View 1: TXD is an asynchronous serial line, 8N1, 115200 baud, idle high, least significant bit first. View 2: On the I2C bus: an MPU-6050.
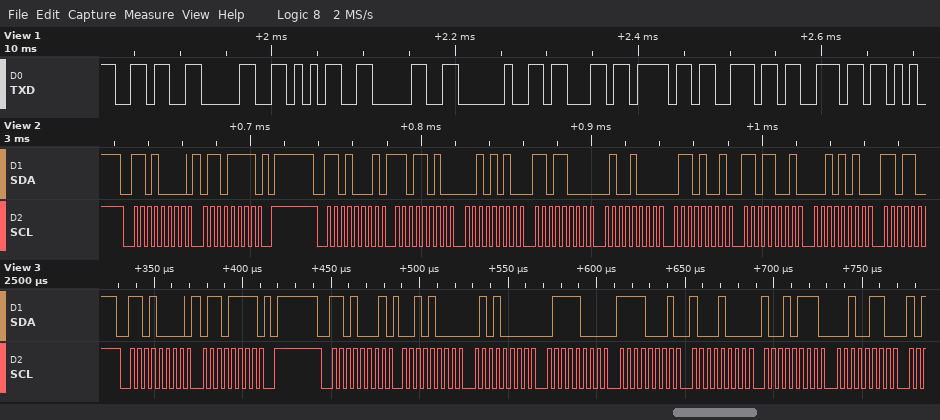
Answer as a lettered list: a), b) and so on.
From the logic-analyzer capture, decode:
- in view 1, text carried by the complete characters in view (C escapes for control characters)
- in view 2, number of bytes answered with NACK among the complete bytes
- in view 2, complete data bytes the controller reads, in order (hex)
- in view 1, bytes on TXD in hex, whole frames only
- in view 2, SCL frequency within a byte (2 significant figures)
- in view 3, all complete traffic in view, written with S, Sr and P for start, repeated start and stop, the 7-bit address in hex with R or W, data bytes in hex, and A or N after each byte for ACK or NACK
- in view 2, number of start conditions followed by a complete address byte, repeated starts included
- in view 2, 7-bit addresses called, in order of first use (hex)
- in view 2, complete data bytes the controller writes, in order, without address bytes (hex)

a) "6050 conn"
b) 0
c) DA 2A D8 48 69 D9 2A
d) 36 30 35 30 20 63 6F 6E 6E
e) 250 kHz
f) S 68W A 6F A P S 68R A 28 A 50 A 78 A F1 A 88 A 97 A 26 A
g) 2
h) 0x68
i) 6F
